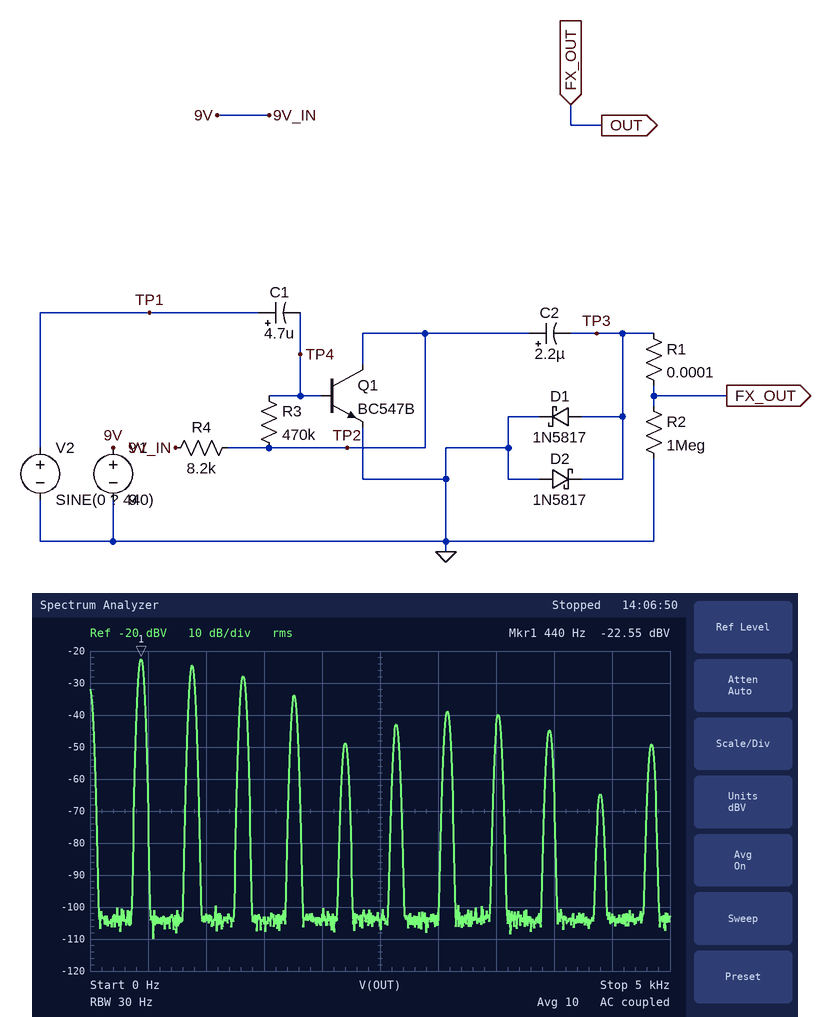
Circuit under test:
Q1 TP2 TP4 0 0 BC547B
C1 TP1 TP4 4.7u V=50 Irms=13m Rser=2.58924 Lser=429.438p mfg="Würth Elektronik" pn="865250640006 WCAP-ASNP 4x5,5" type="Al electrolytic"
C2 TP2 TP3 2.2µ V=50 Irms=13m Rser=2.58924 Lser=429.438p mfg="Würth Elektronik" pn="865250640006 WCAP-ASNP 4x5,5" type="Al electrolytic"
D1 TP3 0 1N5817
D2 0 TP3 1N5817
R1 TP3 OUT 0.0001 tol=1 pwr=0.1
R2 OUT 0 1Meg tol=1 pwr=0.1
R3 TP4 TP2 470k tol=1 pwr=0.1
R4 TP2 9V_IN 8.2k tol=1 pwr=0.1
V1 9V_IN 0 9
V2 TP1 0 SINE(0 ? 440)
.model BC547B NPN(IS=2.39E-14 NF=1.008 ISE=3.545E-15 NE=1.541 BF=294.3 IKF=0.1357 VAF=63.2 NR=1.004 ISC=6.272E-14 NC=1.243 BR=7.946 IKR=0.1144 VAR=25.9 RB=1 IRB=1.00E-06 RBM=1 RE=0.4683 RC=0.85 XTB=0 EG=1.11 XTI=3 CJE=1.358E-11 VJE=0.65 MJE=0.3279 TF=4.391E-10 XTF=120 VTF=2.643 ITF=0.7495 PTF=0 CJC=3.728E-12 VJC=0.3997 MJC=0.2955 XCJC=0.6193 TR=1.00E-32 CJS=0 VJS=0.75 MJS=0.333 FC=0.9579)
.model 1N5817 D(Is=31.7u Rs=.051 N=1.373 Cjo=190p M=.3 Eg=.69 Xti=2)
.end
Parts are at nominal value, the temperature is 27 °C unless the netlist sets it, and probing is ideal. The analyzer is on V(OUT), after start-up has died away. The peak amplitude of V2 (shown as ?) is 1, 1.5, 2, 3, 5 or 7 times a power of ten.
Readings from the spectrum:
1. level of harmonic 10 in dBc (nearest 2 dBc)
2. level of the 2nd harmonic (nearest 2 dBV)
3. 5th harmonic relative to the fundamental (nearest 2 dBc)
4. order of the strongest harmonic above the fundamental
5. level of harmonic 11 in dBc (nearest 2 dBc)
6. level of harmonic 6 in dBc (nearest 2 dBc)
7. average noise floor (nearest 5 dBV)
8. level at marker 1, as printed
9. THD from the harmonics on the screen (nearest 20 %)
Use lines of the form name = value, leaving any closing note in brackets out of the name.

level of harmonic 10 in dBc = -42 dBc
level of the 2nd harmonic = -24 dBV
5th harmonic relative to the fundamental = -26 dBc
order of the strongest harmonic above the fundamental = 2
level of harmonic 11 in dBc = -26 dBc
level of harmonic 6 in dBc = -20 dBc
average noise floor = -105 dBV
level at marker 1, as printed = -22.55 dBV
THD from the harmonics on the screen = 100 %
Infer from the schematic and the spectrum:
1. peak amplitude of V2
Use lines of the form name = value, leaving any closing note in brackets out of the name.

peak amplitude of V2 = 300 mV
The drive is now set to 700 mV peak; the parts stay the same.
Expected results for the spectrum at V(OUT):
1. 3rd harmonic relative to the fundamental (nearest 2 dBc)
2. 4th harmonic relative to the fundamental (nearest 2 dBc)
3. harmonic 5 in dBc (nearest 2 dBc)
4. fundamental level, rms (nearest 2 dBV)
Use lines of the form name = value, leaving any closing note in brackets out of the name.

3rd harmonic relative to the fundamental = -2 dBc
4th harmonic relative to the fundamental = -4 dBc
harmonic 5 in dBc = -8 dBc
fundamental level, rms = -24 dBV
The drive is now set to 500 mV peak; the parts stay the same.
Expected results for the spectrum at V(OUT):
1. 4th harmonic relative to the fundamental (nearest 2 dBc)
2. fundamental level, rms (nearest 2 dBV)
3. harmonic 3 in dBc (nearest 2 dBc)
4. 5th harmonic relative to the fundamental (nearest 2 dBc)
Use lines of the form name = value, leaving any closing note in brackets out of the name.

4th harmonic relative to the fundamental = -6 dBc
fundamental level, rms = -24 dBV
harmonic 3 in dBc = -4 dBc
5th harmonic relative to the fundamental = -12 dBc
